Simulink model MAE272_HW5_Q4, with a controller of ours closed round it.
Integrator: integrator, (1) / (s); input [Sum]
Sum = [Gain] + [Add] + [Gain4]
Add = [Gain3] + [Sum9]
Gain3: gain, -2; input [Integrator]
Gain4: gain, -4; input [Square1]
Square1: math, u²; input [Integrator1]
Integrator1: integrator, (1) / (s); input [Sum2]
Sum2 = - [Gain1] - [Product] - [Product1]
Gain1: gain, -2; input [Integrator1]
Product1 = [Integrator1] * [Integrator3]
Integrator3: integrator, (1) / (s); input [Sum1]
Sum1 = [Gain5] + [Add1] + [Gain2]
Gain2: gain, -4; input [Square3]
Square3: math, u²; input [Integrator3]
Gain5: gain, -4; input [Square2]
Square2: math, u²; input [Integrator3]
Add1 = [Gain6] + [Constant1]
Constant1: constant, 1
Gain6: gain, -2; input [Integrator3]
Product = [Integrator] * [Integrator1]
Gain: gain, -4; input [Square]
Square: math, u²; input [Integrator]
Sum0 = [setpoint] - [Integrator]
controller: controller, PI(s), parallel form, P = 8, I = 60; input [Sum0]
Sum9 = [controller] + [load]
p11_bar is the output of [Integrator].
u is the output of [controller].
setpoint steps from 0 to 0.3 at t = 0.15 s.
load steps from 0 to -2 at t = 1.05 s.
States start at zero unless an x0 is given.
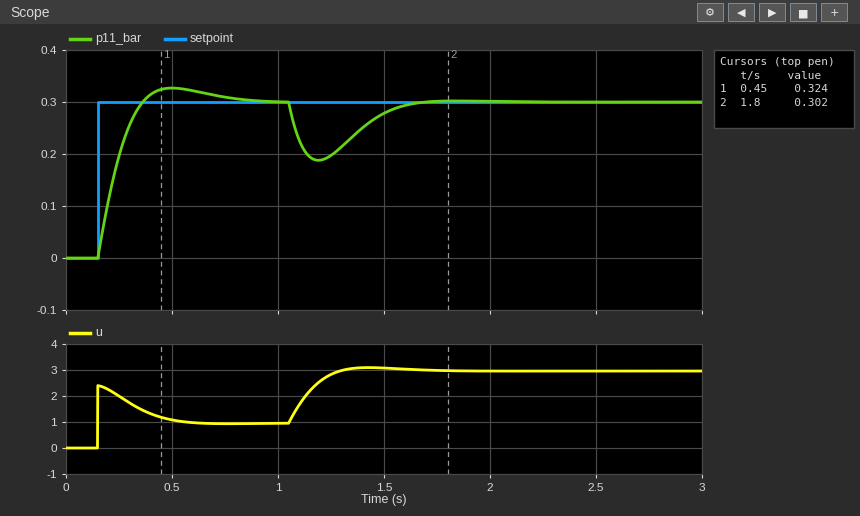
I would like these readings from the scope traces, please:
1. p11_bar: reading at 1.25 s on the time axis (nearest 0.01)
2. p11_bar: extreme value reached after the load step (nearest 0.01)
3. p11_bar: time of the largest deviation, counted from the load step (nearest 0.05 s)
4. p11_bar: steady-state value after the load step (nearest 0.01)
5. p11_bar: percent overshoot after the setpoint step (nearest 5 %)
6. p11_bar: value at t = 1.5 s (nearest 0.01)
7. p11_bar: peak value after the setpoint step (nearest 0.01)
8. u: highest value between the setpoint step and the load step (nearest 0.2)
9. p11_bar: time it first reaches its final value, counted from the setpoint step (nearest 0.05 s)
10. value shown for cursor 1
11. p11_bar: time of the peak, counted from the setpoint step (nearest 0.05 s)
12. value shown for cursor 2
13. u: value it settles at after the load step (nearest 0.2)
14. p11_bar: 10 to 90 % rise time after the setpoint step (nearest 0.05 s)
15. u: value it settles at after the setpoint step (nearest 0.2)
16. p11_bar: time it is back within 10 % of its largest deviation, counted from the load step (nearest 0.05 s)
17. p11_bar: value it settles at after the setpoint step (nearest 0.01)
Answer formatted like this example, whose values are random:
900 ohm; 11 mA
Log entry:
0.20; 0.19; 0.15 s; 0.30; 10 %; 0.28; 0.33; 2.4; 0.20 s; 0.324; 0.35 s; 0.302; 3.0; 0.15 s; 1.0; 0.50 s; 0.30
